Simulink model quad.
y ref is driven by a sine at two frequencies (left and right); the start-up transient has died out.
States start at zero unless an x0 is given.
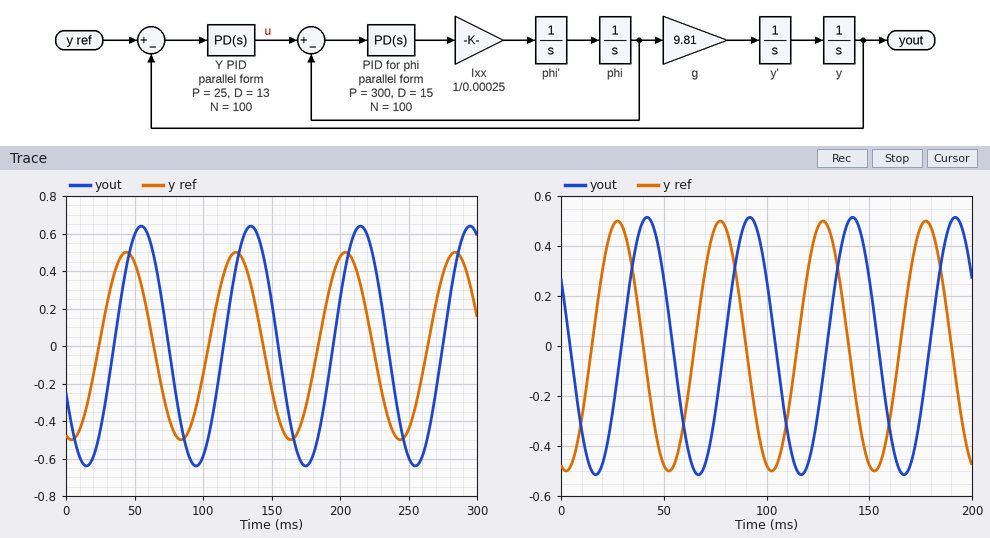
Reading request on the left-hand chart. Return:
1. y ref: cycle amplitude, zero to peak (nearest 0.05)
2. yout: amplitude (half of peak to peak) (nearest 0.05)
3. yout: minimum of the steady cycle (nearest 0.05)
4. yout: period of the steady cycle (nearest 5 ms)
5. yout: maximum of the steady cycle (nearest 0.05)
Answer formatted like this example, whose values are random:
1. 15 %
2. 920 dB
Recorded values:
1. 0.50
2. 0.65
3. -0.65
4. 80 ms
5. 0.65
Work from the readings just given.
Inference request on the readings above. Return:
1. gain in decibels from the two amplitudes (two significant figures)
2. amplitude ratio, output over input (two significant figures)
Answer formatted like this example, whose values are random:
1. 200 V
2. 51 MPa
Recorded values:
1. 2.3 dB
2. 1.3
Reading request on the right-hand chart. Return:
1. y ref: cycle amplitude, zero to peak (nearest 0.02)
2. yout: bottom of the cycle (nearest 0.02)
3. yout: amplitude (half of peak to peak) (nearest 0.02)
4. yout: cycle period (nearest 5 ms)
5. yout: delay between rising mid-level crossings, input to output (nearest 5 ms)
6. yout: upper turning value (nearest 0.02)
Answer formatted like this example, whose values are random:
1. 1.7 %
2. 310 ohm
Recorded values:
1. 0.50
2. -0.52
3. 0.52
4. 50 ms
5. 15 ms
6. 0.52
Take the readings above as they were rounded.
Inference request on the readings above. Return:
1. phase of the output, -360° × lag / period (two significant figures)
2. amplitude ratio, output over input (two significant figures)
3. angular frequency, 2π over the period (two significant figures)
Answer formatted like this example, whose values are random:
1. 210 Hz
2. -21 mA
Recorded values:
1. -110°
2. 1.0
3. 0.13 rad/ms
